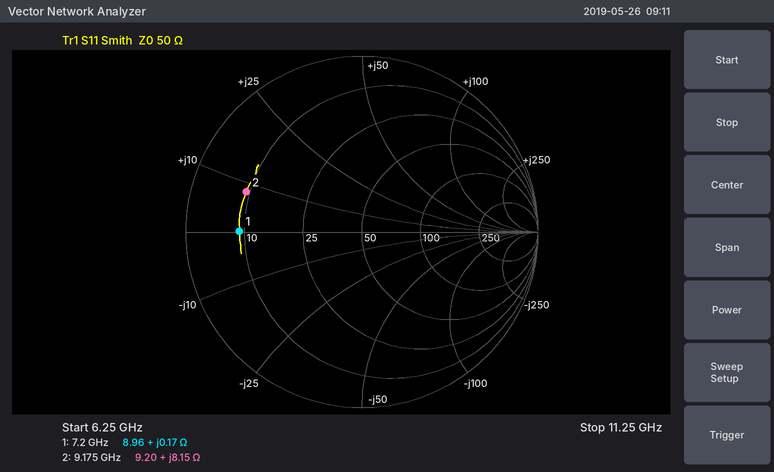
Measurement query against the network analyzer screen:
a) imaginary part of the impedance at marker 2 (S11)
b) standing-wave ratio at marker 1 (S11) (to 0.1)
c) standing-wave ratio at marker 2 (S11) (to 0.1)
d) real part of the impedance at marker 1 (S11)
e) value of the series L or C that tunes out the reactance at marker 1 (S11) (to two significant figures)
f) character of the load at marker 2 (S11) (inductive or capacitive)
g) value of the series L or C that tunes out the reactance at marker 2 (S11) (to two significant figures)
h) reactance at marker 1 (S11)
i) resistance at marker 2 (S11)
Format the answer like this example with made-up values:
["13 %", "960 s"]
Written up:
["+8.15 Ω", "5.6", "5.6", "8.96 Ω", "130 pF", "inductive", "2.1 pF", "+0.17 Ω", "9.20 Ω"]
